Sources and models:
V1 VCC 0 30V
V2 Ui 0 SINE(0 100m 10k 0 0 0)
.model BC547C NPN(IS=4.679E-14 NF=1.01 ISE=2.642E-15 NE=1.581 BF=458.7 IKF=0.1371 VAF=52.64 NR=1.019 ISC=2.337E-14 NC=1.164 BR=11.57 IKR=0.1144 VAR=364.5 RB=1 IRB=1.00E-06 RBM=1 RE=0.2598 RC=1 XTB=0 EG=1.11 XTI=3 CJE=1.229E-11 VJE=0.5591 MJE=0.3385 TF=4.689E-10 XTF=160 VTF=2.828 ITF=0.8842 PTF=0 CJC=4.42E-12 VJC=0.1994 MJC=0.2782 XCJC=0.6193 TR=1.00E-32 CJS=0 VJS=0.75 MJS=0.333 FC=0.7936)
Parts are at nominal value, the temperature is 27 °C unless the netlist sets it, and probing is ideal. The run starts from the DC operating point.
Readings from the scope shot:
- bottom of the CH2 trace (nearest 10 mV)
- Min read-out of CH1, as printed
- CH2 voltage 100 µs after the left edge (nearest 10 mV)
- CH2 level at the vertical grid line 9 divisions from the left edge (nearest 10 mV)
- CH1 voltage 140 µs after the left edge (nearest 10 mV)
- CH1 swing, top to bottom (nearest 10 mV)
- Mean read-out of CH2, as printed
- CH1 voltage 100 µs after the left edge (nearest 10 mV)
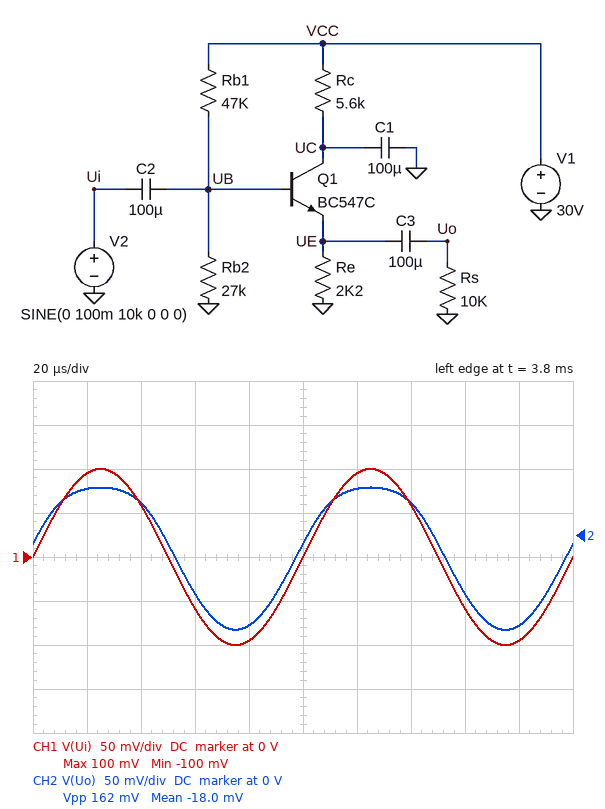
-110 mV
-100 mV
-10 mV
-100 mV
60 mV
200 mV
-18.0 mV
0 V
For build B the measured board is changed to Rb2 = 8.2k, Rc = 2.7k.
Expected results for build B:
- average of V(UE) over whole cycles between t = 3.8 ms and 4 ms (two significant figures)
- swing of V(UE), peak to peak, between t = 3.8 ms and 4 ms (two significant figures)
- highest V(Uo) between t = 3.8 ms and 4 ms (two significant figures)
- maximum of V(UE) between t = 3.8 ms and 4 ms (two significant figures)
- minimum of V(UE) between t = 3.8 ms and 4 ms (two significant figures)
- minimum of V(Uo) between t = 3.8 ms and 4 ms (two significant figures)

3.8 V
200 mV
99 mV
3.9 V
3.7 V
-99 mV
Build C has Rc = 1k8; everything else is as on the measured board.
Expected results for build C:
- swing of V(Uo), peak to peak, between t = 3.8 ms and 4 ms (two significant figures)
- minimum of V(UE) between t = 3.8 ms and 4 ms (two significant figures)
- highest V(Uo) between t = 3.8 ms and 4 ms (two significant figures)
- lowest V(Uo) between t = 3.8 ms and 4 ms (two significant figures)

200 mV
10 V
100 mV
-100 mV
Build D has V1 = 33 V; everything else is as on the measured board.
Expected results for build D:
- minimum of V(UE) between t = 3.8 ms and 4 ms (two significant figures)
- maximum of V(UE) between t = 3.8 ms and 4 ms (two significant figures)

9.4 V
9.5 V
